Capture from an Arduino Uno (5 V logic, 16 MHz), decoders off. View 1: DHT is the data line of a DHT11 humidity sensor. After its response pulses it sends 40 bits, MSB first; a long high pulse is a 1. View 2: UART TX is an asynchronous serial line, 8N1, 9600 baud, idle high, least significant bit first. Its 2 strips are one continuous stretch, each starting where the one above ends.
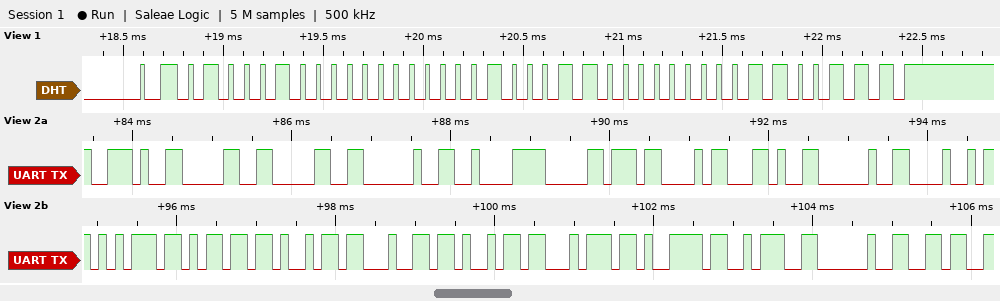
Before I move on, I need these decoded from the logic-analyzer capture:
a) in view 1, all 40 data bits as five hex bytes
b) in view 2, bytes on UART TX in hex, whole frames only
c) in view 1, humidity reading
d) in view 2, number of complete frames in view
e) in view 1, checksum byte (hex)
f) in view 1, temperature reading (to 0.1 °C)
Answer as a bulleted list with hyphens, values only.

- 44 00 23 00 67
- 2E 30 30 20 C2 B0 43 2C 20 48 75 6D 69 64 69 74 79 3A 20 36
- 68 %
- 20
- 0x67
- 35.0 °C
